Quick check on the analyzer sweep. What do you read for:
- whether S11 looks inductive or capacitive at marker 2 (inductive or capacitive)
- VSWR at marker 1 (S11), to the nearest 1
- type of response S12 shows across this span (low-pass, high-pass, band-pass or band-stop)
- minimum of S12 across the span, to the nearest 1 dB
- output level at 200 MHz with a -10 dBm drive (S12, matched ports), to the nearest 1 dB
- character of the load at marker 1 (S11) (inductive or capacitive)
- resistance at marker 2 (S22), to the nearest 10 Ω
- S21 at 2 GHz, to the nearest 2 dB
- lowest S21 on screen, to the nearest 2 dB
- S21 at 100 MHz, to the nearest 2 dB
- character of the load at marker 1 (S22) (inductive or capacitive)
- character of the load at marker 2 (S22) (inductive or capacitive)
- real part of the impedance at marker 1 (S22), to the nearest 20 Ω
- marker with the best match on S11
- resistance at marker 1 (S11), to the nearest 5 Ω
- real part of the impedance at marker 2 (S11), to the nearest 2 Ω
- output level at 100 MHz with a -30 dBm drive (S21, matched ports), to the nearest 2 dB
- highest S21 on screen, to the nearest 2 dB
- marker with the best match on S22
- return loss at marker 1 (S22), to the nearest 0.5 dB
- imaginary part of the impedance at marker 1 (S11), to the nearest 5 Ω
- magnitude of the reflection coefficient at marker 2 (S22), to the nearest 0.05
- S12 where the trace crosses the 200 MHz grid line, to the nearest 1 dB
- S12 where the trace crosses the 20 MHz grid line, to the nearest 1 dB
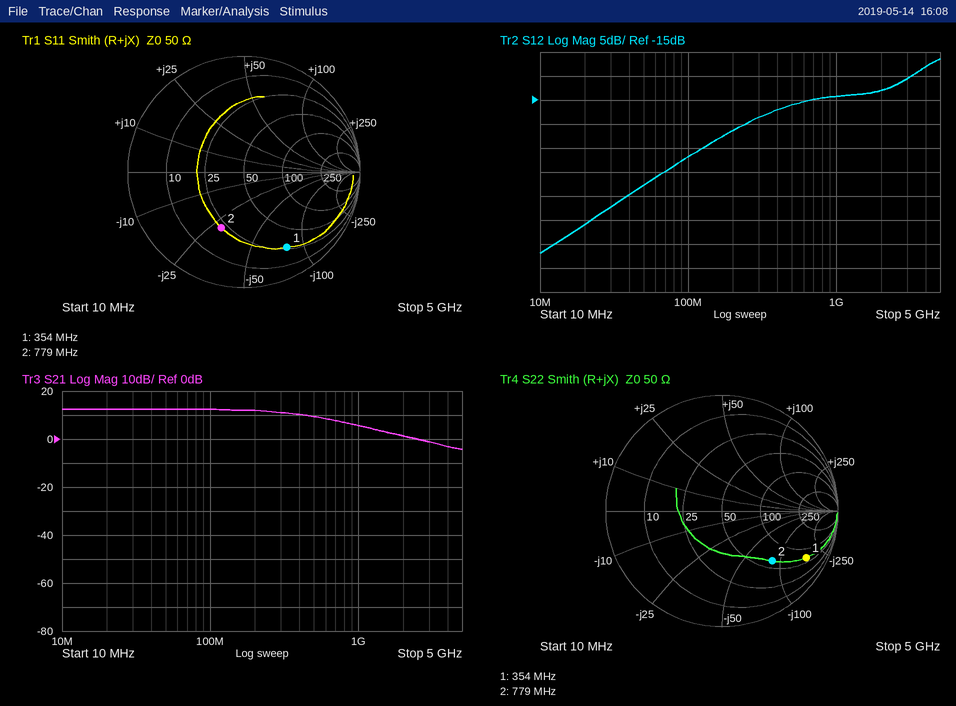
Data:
capacitive
7
high-pass
-47 dB
-31 dBm
capacitive
60 Ω
2 dB
-4 dB
12 dB
capacitive
capacitive
60 Ω
marker 2
25 Ω
22 Ω
-18 dBm
12 dB
marker 2
1.5 dB
-80 Ω
0.60
-21 dB
-41 dB
